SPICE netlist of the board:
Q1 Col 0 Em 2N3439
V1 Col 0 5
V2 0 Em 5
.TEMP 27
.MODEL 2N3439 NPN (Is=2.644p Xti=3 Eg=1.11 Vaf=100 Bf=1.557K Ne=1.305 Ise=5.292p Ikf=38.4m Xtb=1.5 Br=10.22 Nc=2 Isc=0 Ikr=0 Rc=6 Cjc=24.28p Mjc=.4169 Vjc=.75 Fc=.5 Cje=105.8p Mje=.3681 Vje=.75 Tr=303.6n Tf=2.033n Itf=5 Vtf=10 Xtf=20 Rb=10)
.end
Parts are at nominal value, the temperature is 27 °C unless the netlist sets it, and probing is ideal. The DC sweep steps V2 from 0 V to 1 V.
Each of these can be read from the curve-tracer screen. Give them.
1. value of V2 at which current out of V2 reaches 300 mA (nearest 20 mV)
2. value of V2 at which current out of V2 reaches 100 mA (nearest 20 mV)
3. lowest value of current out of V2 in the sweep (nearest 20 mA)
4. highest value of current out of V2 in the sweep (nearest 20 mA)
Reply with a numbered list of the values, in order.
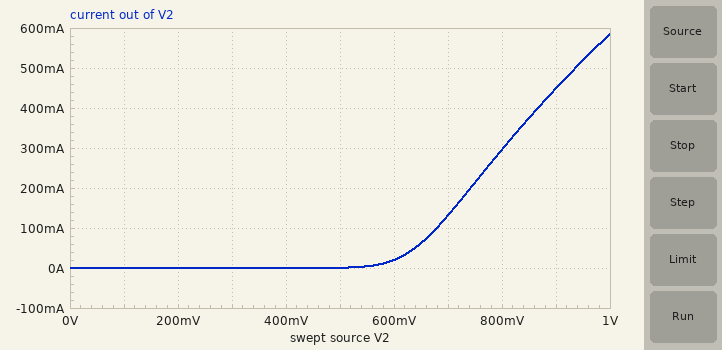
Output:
1. 800 mV
2. 680 mV
3. 0 A
4. 580 mA
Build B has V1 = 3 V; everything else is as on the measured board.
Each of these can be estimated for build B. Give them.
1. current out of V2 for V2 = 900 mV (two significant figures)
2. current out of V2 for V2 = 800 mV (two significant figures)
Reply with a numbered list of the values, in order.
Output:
1. 440 mA
2. 290 mA
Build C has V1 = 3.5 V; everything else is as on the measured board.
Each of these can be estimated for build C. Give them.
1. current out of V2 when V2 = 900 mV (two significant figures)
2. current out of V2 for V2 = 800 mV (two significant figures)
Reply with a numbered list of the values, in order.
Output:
1. 440 mA
2. 290 mA
